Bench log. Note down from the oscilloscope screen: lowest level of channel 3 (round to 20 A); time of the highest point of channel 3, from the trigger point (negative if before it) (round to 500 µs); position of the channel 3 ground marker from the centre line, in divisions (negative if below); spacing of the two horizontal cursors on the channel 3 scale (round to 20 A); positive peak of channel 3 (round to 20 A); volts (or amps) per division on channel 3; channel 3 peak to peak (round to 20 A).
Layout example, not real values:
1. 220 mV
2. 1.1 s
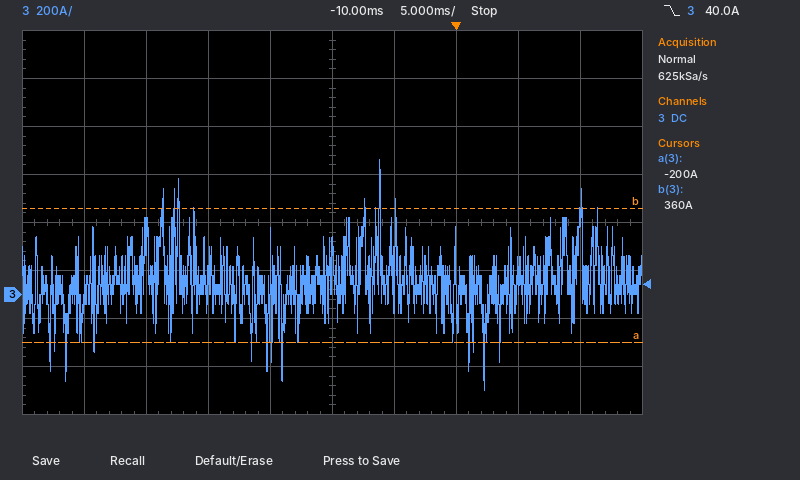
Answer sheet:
1. -400 A
2. -6.0 ms
3. -1.5 div
4. 560 A
5. 560 A
6. 200 A
7. 960 A
